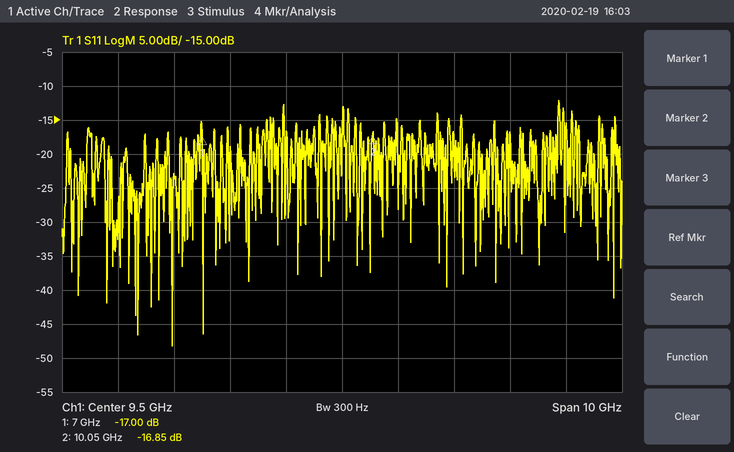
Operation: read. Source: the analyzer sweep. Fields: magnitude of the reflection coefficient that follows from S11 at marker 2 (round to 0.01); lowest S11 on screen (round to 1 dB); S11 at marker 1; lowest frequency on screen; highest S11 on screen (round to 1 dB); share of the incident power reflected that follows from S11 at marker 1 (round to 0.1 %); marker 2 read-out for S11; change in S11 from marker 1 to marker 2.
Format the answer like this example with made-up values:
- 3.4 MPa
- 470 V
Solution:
- 0.14
- -48 dB
- -17.00 dB
- 4.5 GHz
- -12 dB
- 2.0 %
- -16.85 dB
- 0.15 dB
